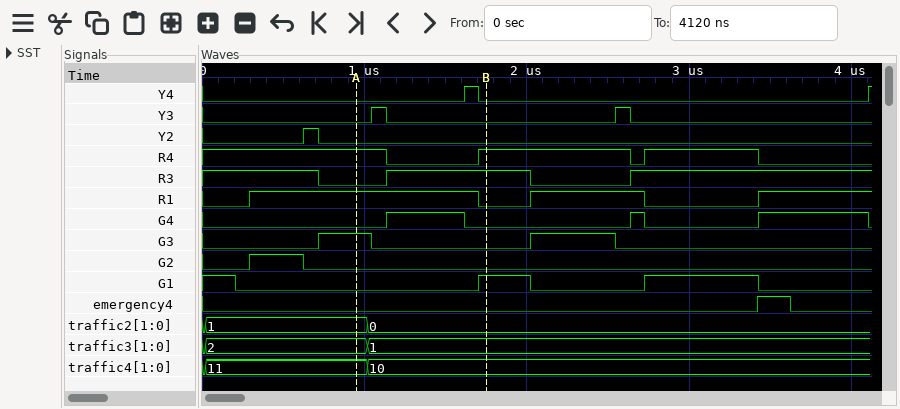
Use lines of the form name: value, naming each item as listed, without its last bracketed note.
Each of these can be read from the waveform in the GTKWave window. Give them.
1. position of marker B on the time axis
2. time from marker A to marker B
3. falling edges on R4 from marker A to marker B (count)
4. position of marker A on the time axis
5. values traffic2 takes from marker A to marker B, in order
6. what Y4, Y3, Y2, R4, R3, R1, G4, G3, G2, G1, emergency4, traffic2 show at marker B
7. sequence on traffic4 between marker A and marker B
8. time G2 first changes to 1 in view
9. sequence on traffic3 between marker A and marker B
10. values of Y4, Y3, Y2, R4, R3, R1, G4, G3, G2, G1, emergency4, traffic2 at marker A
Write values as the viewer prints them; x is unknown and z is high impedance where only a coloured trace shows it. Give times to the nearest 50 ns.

position of marker B on the time axis: 1750 ns
time from marker A to marker B: 800 ns
falling edges on R4 from marker A to marker B: 1
position of marker A on the time axis: 950 ns
values traffic2 takes from marker A to marker B, in order: 1, 0
what Y4, Y3, Y2, R4, R3, R1, G4, G3, G2, G1, emergency4, traffic2 show at marker B: Y4=0, Y3=0, Y2=0, R4=1, R3=1, R1=0, G4=0, G3=0, G2=0, G1=1, emergency4=0, traffic2=0
sequence on traffic4 between marker A and marker B: 11, 10
time G2 first changes to 1 in view: 300 ns
sequence on traffic3 between marker A and marker B: 2, 1
values of Y4, Y3, Y2, R4, R3, R1, G4, G3, G2, G1, emergency4, traffic2 at marker A: Y4=0, Y3=0, Y2=0, R4=1, R3=0, R1=1, G4=0, G3=1, G2=0, G1=0, emergency4=0, traffic2=1
